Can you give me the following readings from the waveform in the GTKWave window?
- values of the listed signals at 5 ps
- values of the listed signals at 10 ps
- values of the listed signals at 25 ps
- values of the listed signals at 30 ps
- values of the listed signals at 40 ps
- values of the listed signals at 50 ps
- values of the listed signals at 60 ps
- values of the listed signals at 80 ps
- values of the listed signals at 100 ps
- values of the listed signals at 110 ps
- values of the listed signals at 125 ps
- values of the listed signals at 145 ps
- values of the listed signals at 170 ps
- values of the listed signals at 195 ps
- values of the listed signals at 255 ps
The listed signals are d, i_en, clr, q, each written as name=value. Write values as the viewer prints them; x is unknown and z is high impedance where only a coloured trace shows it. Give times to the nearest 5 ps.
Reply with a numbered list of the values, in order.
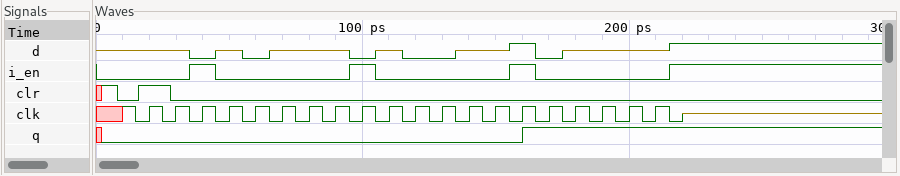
1. d=z, i_en=0, clr=1, q=0
2. d=z, i_en=0, clr=0, q=0
3. d=z, i_en=0, clr=1, q=0
4. d=z, i_en=0, clr=0, q=0
5. d=0, i_en=1, clr=0, q=0
6. d=z, i_en=0, clr=0, q=0
7. d=0, i_en=0, clr=0, q=0
8. d=z, i_en=0, clr=0, q=0
9. d=0, i_en=1, clr=0, q=0
10. d=z, i_en=0, clr=0, q=0
11. d=0, i_en=0, clr=0, q=0
12. d=z, i_en=0, clr=0, q=0
13. d=0, i_en=0, clr=0, q=1
14. d=z, i_en=0, clr=0, q=1
15. d=1, i_en=1, clr=0, q=1
